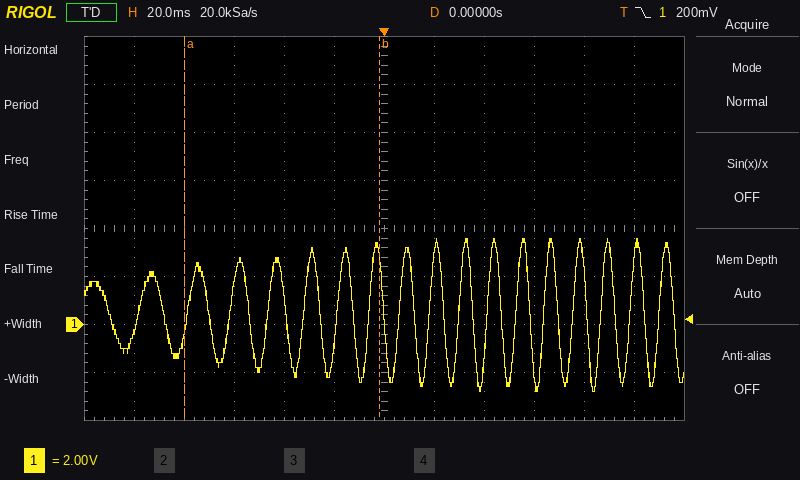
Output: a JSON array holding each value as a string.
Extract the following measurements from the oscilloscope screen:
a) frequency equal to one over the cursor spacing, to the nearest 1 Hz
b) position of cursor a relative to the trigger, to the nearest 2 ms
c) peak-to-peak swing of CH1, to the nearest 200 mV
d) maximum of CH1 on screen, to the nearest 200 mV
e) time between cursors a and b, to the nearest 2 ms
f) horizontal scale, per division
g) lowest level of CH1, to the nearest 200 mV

["13 Hz", "-80 ms", "6.4 V", "3.6 V", "78 ms", "20 ms", "-2.8 V"]
